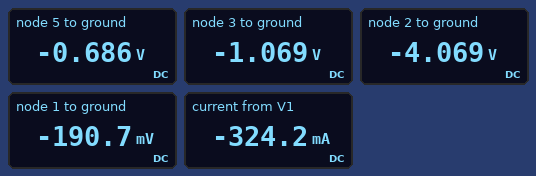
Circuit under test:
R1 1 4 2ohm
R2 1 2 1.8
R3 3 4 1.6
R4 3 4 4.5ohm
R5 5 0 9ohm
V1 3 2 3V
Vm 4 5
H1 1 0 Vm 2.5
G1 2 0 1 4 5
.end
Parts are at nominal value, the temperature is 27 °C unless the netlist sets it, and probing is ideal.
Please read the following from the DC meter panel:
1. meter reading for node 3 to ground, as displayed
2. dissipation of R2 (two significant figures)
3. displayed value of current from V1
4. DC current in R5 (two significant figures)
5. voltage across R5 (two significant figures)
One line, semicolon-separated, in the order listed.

-1.069 V; 8.4 W; -324.2 mA; 76 mA; 690 mV
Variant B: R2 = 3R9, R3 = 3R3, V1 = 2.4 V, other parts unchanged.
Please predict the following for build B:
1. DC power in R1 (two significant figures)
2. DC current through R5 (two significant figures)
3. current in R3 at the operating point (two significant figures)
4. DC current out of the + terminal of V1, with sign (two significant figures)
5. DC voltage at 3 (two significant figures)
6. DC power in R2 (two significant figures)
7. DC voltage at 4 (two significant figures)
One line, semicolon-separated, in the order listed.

13 mW; 25 mA; 62 mA; -110 mA; -430 mV; 2.0 W; -230 mV
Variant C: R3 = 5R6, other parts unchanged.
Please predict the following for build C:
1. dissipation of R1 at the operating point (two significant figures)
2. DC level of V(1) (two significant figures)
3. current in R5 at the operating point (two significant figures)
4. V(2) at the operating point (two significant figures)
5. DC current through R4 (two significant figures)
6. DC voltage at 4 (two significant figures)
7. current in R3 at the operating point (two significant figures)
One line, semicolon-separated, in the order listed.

170 mW; -220 mV; 89 mA; -4.7 V; 210 mA; -800 mV; 170 mA
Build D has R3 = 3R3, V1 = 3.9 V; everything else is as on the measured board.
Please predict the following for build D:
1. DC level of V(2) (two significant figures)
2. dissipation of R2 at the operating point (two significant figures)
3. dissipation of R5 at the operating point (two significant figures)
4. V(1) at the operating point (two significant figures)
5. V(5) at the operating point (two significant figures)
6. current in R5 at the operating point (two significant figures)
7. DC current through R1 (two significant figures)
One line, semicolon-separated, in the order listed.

-5.7 V; 17 W; 100 mW; -270 mV; -970 mV; 110 mA; 350 mA
